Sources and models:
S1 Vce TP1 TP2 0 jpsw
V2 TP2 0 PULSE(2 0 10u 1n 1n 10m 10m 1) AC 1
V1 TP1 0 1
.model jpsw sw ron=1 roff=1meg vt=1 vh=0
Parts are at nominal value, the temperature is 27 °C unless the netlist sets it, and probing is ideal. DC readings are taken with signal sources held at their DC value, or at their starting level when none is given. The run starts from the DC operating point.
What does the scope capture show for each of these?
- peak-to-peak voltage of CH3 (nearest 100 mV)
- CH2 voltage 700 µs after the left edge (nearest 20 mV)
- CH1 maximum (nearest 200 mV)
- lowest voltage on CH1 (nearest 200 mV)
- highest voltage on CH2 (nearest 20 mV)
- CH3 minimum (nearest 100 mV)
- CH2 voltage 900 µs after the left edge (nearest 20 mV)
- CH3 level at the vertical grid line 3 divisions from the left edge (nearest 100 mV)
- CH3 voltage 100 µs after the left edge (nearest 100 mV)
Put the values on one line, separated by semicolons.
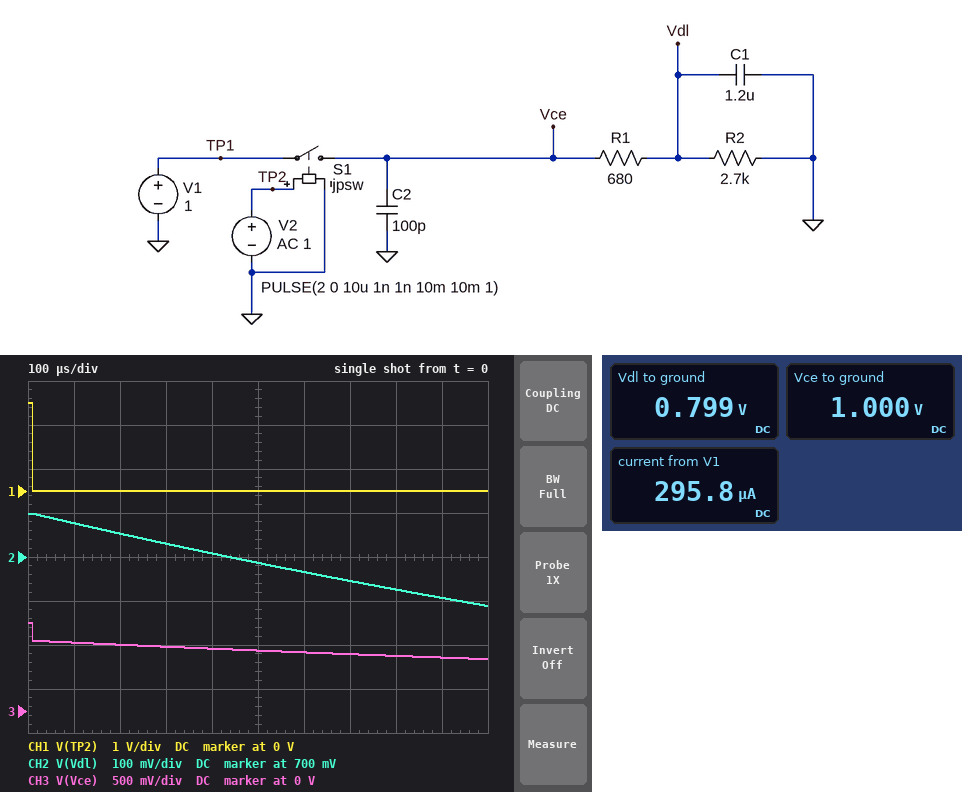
400 mV; 640 mV; 2.0 V; 0 V; 800 mV; 600 mV; 600 mV; 700 mV; 800 mV
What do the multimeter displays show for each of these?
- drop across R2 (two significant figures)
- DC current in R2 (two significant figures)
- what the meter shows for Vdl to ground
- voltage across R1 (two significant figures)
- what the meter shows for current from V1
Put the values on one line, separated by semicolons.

800 mV; 300 µA; 0.799 V; 200 mV; 295.8 µA
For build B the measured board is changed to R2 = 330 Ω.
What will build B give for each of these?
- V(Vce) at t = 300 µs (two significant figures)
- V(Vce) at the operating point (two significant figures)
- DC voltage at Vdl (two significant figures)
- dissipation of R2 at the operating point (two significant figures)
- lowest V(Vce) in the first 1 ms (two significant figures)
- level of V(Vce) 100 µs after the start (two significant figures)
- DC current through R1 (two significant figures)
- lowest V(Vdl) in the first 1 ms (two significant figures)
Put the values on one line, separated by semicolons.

160 mV; 1.0 V; 330 mV; 320 µW; 28 mV; 260 mV; 990 µA; 27 mV
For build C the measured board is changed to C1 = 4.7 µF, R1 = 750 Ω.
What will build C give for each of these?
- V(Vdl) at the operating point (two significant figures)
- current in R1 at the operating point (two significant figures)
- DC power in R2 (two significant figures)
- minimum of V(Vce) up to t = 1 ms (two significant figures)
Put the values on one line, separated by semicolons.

780 mV; 290 µA; 230 µW; 720 mV
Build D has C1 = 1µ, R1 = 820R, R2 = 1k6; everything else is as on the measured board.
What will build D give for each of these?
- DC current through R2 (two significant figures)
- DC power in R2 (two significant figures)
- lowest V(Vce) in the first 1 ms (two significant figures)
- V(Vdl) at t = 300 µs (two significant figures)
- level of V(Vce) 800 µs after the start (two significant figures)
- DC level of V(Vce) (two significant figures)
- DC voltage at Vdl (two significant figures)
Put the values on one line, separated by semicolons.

410 µA; 270 µW; 360 mV; 550 mV; 400 mV; 1.0 V; 660 mV
